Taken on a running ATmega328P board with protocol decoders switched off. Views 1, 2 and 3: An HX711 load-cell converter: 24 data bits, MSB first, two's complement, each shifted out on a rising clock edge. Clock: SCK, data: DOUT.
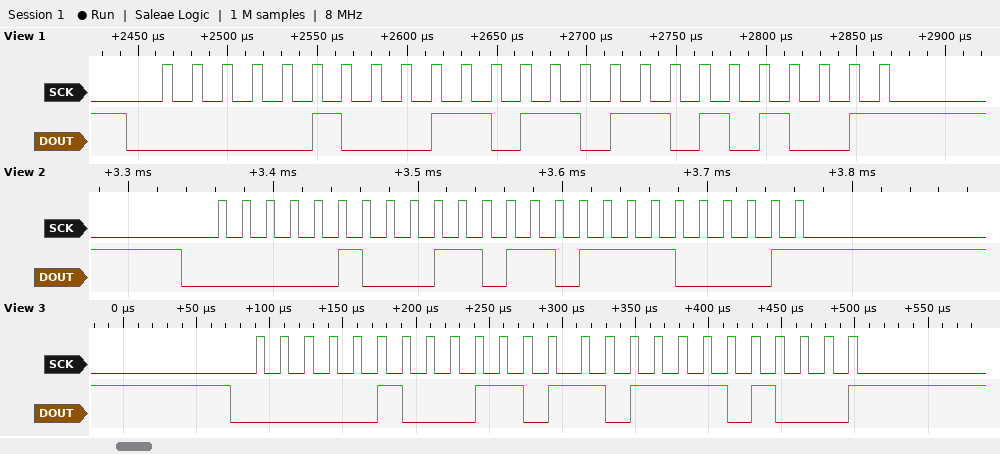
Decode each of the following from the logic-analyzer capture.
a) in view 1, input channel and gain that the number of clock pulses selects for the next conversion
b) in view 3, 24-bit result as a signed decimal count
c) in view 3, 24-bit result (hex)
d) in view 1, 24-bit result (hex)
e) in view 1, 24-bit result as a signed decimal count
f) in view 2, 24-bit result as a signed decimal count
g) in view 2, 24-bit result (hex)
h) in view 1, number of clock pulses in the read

channel A, gain 128
290280
0x046DE8
0x046DA9
290217
290273
0x046DE1
25
